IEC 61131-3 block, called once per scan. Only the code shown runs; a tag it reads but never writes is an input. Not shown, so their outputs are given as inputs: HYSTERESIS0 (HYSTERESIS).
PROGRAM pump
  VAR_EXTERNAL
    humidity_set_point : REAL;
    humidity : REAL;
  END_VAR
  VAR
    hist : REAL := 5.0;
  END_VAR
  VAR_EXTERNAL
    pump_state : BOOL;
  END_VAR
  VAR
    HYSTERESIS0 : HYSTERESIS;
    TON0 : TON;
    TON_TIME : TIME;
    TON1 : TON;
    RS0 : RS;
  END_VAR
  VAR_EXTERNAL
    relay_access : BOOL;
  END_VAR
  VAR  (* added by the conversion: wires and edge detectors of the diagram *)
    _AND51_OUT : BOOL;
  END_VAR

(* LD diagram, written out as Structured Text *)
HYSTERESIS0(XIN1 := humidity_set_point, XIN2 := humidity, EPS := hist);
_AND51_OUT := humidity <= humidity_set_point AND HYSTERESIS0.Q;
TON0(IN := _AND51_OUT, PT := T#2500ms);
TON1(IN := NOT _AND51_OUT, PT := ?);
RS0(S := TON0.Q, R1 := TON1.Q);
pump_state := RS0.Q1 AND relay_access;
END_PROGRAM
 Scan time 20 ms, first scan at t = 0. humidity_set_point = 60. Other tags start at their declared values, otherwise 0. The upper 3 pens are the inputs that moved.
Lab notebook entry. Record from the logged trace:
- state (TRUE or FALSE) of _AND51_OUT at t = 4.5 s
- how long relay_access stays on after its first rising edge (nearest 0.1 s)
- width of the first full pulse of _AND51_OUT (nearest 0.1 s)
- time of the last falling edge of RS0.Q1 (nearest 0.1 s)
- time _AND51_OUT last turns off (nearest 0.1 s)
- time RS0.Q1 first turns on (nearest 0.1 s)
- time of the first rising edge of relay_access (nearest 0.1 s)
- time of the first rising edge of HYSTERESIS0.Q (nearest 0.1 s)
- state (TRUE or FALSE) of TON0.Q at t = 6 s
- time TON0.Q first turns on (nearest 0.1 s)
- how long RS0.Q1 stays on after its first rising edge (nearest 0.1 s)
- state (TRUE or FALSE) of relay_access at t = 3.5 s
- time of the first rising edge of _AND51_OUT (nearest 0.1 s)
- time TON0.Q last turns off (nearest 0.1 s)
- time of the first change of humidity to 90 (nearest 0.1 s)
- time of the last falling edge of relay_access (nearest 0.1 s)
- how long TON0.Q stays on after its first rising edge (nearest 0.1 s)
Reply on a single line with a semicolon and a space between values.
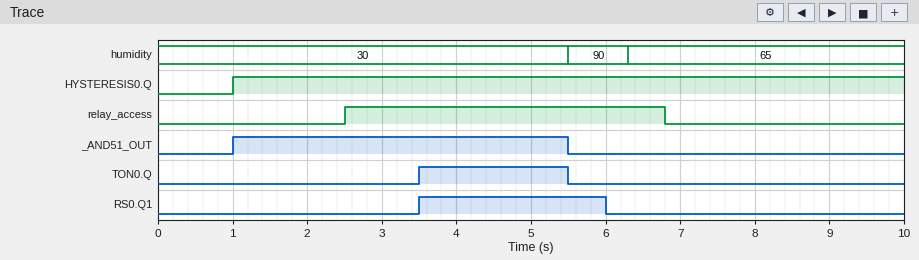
TRUE; 4.3 s; 4.5 s; 6.0 s; 5.5 s; 3.5 s; 2.5 s; 1.0 s; FALSE; 3.5 s; 2.5 s; TRUE; 1.0 s; 5.5 s; 5.5 s; 6.8 s; 2.0 s
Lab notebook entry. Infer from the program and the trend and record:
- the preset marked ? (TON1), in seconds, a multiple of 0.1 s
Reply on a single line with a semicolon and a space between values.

0.5 s
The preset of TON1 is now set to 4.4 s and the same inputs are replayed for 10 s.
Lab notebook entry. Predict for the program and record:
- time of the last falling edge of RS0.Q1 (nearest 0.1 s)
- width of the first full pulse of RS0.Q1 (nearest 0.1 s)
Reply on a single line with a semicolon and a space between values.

9.9 s; 6.4 s
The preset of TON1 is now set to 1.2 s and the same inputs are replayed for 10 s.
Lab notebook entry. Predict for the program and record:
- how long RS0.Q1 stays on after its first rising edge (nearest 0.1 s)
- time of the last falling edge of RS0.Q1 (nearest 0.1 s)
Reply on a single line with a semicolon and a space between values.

3.2 s; 6.7 s
